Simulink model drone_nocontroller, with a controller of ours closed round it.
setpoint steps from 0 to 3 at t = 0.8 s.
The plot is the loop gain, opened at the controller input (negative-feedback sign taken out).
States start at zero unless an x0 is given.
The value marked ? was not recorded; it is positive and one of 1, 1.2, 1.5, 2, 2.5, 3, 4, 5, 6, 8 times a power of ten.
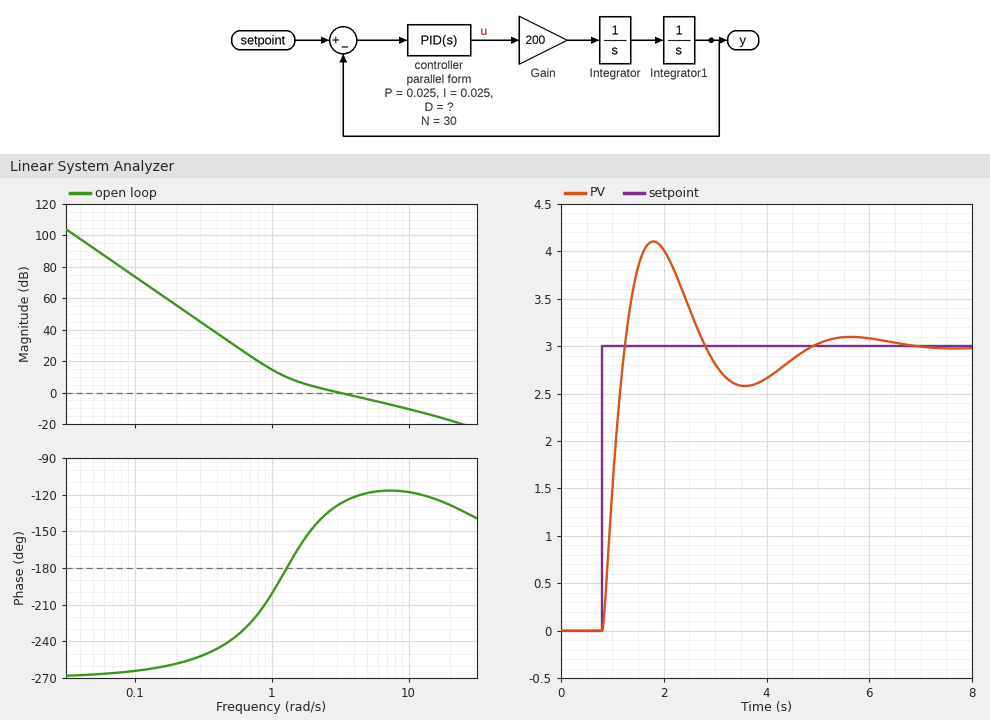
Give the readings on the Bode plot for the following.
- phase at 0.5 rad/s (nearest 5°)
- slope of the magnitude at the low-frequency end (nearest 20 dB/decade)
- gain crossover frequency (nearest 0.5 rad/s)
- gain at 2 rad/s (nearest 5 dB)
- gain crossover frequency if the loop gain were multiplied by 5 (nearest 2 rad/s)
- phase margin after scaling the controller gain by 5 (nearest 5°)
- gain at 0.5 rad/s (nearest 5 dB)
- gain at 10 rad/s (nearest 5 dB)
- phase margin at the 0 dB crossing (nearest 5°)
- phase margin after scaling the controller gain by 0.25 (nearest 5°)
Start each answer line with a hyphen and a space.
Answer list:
- -240°
- -60 dB/decade
- 3.0 rad/s
- 5 dB
- 14 rad/s
- 60°
- 30 dB
- -10 dB
- 50°
- -10°
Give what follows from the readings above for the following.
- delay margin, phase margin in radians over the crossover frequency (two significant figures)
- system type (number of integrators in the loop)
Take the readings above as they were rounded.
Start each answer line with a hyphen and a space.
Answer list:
- 0.29 s
- 3
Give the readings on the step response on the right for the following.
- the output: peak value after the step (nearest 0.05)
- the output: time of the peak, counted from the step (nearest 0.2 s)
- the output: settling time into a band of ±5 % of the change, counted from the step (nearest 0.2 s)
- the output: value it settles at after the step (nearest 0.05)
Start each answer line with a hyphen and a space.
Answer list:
- 4.10
- 1.0 s
- 3.6 s
- 3.00
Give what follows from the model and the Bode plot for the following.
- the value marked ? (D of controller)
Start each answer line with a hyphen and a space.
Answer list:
- 0.015
